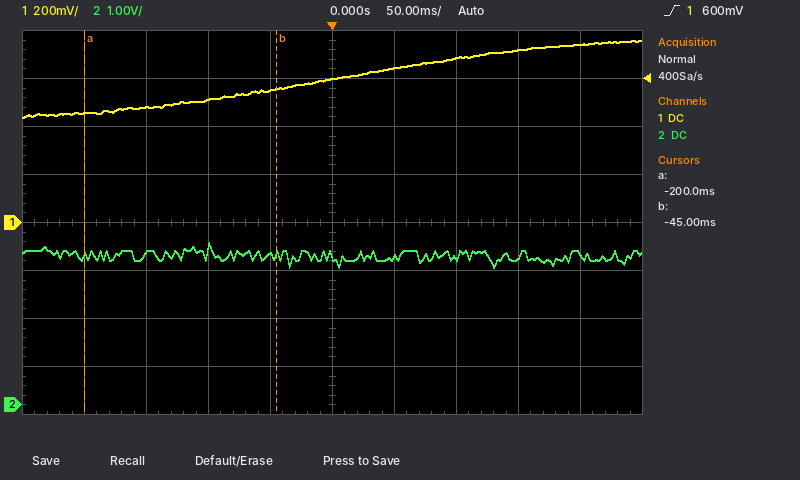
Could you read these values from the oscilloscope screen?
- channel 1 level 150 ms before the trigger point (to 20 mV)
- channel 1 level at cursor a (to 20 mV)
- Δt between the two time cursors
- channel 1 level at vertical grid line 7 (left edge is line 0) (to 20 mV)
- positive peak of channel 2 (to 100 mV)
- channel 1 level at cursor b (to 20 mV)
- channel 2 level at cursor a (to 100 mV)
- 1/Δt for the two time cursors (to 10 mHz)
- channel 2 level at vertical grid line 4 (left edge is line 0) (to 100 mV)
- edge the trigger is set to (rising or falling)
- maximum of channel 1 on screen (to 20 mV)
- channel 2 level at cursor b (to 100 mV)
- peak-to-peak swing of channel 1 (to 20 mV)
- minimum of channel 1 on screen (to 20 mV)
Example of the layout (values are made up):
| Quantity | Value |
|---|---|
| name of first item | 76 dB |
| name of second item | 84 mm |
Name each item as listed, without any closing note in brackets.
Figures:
| Quantity | Value |
|---|---|
| channel 1 level 150 ms before the trigger point | 480 mV |
| channel 1 level at cursor a | 460 mV |
| Δt between the two time cursors | 155 ms |
| channel 1 level at vertical grid line 7 (left edge is line 0) | 680 mV |
| positive peak of channel 2 | 3.4 V |
| channel 1 level at cursor b | 560 mV |
| channel 2 level at cursor a | 3.1 V |
| 1/Δt for the two time cursors | 6.45 Hz |
| channel 2 level at vertical grid line 4 (left edge is line 0) | 3.1 V |
| edge the trigger is set to | rising |
| maximum of channel 1 on screen | 760 mV |
| channel 2 level at cursor b | 3.1 V |
| peak-to-peak swing of channel 1 | 320 mV |
| minimum of channel 1 on screen | 440 mV |
